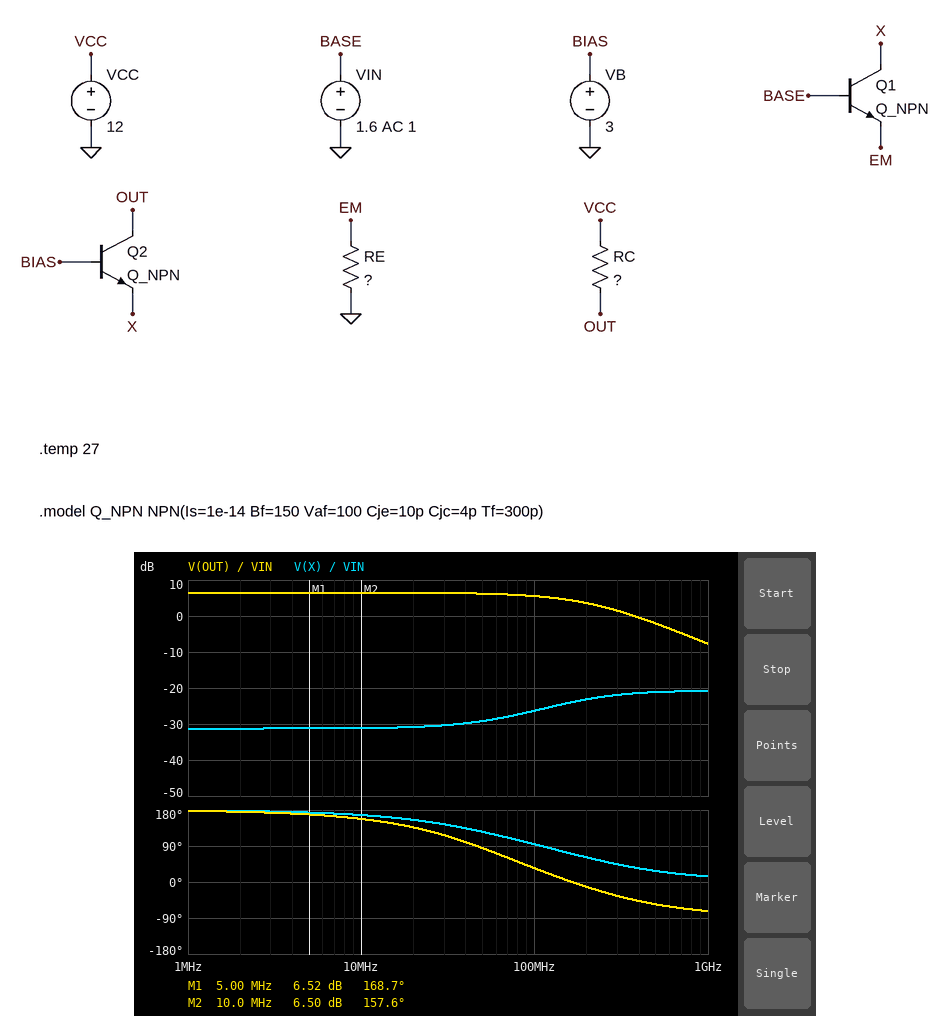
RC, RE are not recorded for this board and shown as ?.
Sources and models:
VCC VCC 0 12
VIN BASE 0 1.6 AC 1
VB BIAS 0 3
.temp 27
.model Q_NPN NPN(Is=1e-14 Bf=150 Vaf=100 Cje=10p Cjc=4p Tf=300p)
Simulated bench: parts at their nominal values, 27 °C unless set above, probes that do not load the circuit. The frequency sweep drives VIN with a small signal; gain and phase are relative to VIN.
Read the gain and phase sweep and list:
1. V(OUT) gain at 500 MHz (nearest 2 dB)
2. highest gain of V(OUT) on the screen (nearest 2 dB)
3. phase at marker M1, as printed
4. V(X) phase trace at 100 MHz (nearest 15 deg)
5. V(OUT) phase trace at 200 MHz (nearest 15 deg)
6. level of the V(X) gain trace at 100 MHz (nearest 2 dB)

-2 dB
6 dB
168.7 deg
90 deg
-15 deg
-26 dB
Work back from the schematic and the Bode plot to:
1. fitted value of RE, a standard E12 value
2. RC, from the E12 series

680 Ω
1.5 kΩ
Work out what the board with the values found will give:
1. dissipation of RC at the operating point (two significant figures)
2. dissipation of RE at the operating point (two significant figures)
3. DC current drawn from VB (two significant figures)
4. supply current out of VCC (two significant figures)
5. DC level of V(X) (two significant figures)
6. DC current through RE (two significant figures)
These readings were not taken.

2.8 mW
1.3 mW
8.5 µA
1.4 mA
2.3 V
1.4 mA
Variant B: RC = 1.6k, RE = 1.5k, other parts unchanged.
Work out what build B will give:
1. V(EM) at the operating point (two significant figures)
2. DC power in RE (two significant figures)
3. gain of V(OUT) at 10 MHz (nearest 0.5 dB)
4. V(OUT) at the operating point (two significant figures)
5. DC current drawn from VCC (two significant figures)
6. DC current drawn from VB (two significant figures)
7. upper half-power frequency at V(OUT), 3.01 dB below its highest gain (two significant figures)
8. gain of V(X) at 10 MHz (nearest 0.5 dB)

960 mV
610 µW
0.5 dB
11 V
630 µA
3.9 µA
210 MHz
-31.0 dB
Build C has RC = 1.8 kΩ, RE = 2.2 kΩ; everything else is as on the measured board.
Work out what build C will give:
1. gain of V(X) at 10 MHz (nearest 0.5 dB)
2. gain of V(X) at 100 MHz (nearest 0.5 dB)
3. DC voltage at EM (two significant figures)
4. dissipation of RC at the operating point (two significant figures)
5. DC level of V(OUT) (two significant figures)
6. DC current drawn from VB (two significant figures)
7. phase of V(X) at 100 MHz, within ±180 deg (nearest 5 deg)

-30.5 dB
-20.0 dB
970 mV
340 µW
11 V
2.7 µA
55 deg
